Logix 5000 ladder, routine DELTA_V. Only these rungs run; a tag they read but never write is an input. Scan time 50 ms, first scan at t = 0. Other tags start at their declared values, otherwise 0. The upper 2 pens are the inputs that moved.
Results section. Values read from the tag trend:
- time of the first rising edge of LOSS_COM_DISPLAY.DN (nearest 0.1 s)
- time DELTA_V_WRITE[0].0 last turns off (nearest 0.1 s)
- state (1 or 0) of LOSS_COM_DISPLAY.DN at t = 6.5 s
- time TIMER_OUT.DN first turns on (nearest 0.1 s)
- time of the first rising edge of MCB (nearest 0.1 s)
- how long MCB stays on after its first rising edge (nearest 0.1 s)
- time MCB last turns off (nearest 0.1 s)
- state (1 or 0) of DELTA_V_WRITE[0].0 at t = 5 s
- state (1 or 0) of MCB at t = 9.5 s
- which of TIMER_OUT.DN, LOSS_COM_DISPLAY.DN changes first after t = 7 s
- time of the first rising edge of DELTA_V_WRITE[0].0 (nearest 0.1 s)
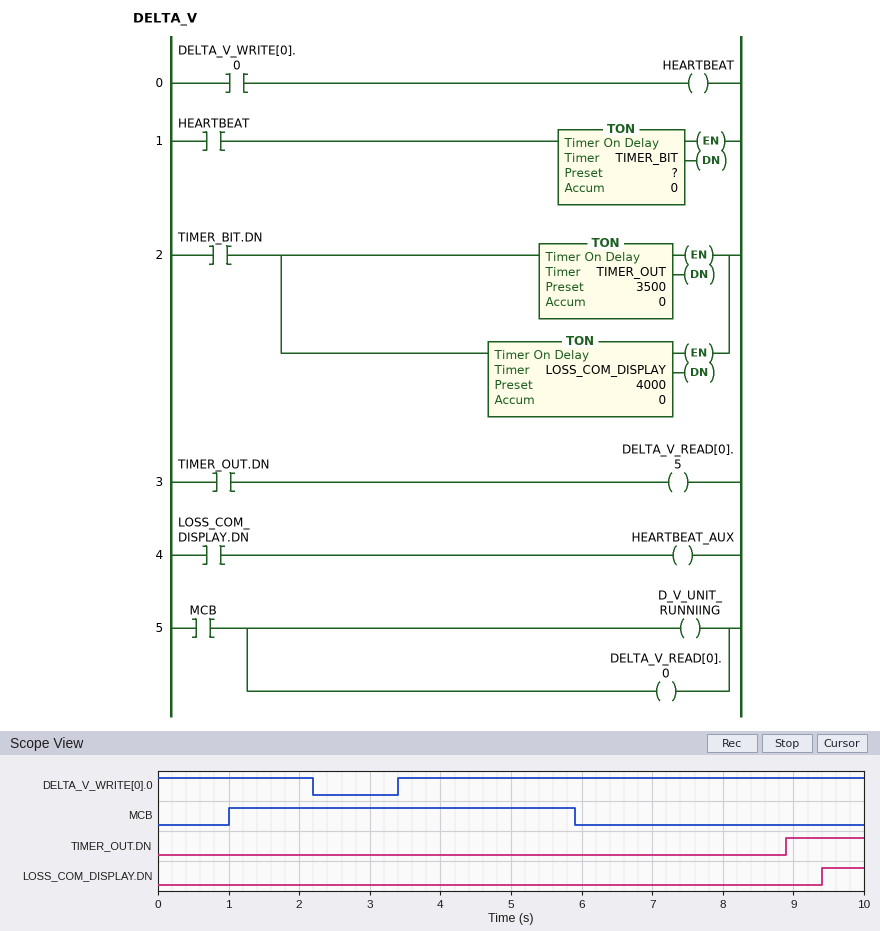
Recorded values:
9.4 s
2.2 s
0
8.9 s
1.0 s
4.9 s
5.9 s
1
0
TIMER_OUT.DN
3.4 s
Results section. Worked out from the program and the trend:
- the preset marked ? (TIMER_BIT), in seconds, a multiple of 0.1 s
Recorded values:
2.0 s
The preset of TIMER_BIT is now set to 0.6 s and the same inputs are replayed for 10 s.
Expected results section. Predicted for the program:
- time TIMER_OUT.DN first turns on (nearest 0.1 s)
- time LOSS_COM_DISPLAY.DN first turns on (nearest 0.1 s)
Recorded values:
7.5 s
8.0 s
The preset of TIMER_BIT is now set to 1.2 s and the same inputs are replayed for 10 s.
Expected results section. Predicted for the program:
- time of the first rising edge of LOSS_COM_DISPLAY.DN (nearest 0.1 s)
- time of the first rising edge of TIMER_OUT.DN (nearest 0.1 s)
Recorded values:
8.6 s
8.1 s
